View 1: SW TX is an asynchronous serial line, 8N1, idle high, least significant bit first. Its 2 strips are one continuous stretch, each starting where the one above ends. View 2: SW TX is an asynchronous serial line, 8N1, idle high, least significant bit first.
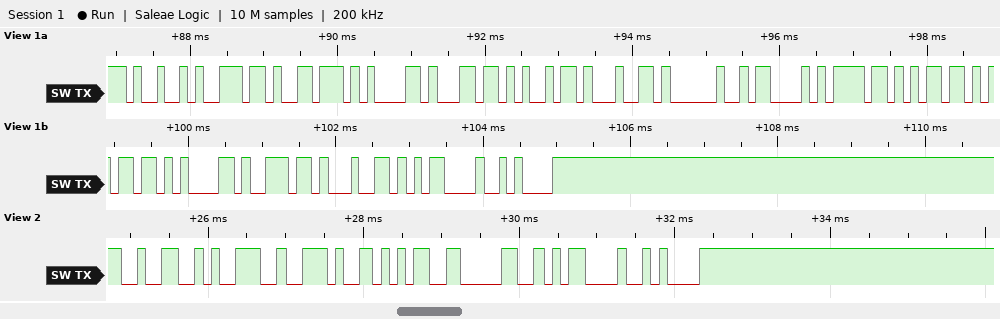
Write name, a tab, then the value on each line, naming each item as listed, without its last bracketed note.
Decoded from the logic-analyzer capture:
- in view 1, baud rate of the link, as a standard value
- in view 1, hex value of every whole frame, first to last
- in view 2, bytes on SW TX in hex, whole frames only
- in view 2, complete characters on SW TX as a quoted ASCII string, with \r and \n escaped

in view 1, baud rate of the link, as a standard value	9600 baud
in view 1, hex value of every whole frame, first to last	49 6E 76 61 6C 69 64 20 43 6F 6D 6D 61 6E 64 0D 0A
in view 2, bytes on SW TX in hex, whole frames only	32 39 2E 35 30 0D 0A
in view 2, complete characters on SW TX as a quoted ASCII string, with \r and \n escaped	"29.50\r\n"
